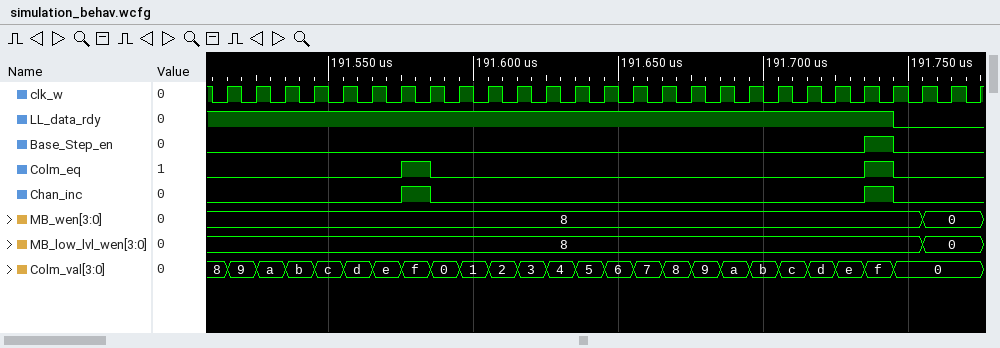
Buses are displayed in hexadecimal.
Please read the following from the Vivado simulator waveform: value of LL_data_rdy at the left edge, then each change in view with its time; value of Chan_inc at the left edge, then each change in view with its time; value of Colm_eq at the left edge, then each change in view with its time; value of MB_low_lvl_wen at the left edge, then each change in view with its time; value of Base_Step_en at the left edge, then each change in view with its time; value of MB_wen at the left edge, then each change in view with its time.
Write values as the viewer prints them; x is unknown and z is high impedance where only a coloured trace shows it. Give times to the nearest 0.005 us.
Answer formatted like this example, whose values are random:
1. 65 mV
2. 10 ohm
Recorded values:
1. 1, 0 at 191.745 us
2. 0, 1 at 191.575 us, 0 at 191.585 us, 1 at 191.735 us, 0 at 191.745 us
3. 0, 1 at 191.575 us, 0 at 191.585 us, 1 at 191.735 us, 0 at 191.745 us
4. 8, 0 at 191.755 us
5. 0, 1 at 191.735 us, 0 at 191.745 us
6. 8, 0 at 191.755 us
